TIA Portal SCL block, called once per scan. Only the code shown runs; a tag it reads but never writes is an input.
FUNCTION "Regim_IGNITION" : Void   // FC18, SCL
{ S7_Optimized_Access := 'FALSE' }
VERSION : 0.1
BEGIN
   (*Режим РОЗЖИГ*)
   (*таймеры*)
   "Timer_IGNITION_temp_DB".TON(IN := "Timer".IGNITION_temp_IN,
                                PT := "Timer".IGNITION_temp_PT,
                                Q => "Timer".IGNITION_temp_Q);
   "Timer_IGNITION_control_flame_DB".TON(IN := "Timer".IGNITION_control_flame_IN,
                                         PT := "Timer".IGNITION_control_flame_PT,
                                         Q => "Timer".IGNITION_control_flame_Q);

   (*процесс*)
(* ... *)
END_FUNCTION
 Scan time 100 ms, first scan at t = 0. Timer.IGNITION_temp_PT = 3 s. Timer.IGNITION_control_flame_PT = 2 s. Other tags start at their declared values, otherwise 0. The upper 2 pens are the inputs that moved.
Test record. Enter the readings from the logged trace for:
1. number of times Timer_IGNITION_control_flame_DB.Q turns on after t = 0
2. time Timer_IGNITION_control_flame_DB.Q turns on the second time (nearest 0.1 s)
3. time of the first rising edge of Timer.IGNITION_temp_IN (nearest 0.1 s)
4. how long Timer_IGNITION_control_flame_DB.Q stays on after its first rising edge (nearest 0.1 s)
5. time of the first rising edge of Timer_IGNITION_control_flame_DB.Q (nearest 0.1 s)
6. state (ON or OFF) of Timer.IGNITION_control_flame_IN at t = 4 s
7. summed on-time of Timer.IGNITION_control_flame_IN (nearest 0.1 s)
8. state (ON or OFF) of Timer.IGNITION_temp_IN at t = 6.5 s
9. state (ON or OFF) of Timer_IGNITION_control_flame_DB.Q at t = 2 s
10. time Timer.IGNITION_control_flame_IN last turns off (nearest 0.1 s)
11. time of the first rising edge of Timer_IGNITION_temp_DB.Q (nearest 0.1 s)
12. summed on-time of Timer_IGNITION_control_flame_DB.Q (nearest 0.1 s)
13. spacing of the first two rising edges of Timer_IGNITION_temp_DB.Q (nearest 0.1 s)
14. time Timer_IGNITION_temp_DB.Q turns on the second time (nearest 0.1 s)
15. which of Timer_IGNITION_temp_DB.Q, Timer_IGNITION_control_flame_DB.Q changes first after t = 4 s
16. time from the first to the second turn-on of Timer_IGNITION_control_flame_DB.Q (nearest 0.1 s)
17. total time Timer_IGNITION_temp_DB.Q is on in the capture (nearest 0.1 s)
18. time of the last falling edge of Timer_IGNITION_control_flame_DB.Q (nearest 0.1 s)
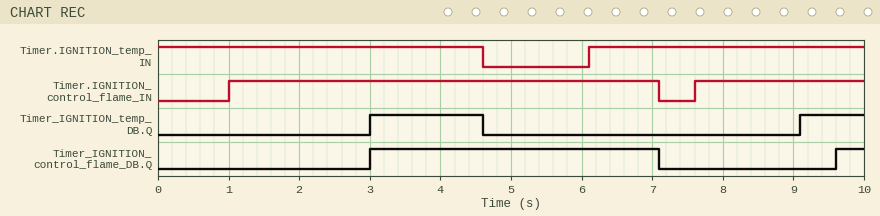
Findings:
2
9.6 s
6.1 s
4.1 s
3.0 s
ON
8.5 s
ON
OFF
7.1 s
3.0 s
4.5 s
6.1 s
9.1 s
Timer_IGNITION_temp_DB.Q
6.6 s
2.5 s
7.1 s
